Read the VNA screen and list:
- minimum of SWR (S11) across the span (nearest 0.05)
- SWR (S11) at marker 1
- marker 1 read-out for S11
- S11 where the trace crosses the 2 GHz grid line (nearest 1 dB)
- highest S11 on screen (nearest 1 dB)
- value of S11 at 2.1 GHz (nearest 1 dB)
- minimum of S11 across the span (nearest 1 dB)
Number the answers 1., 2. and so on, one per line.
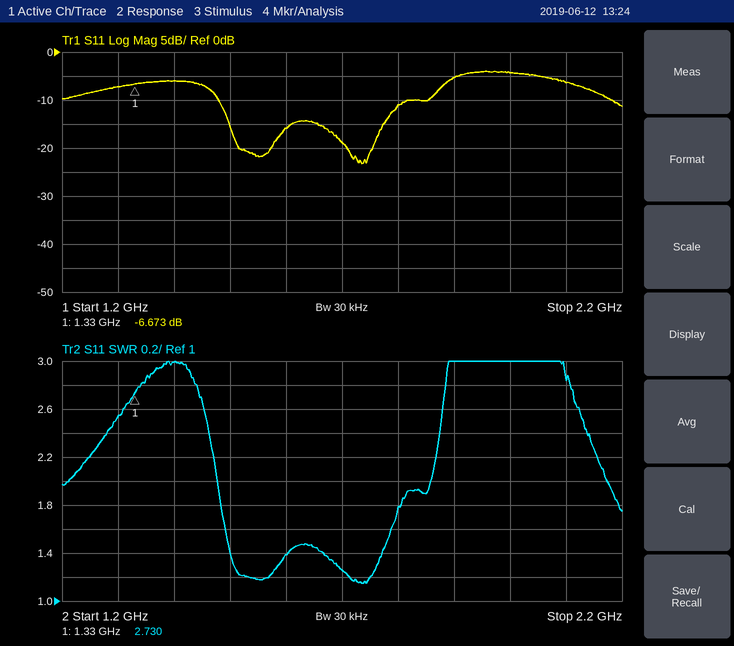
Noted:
1. 1.15
2. 2.730
3. -6.673 dB
4. -4 dB
5. -4 dB
6. -6 dB
7. -23 dB
